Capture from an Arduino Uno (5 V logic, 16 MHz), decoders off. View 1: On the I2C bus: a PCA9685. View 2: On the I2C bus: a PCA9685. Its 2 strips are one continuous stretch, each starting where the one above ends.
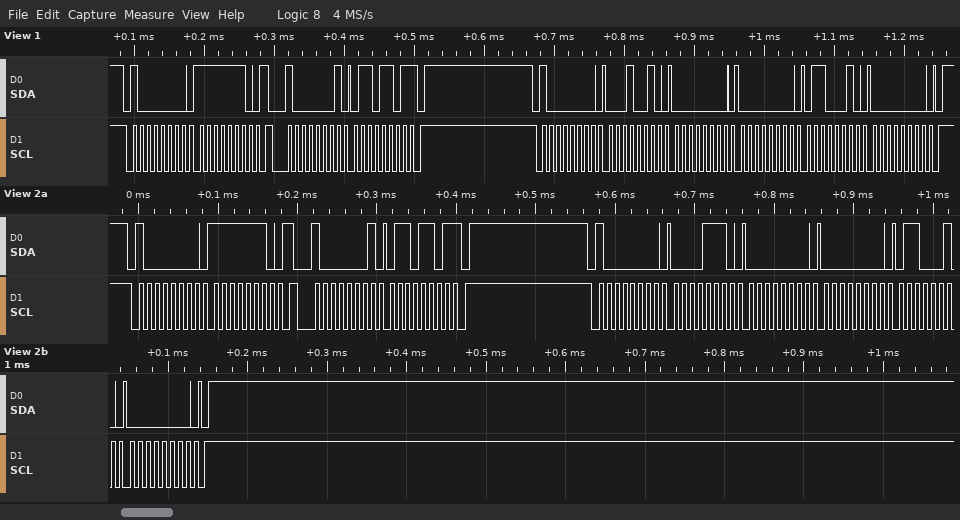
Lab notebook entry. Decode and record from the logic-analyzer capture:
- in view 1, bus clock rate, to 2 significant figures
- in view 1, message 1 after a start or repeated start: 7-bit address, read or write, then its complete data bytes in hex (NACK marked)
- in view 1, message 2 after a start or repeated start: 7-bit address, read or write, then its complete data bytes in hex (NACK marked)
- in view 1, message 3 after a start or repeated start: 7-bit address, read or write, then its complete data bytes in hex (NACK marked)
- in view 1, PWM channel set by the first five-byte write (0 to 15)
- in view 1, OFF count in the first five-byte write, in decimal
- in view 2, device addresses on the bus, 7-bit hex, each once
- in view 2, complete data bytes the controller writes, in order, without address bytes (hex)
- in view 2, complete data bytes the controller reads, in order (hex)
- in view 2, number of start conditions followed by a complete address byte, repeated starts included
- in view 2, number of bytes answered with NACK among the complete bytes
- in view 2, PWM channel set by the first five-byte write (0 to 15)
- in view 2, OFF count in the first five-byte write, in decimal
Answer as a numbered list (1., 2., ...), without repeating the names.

1. 100 kHz
2. 0x40 write: FE
3. 0x40 read: 6D NACK
4. 0x40 write: 12 00 00 62 00
5. 3
6. 98
7. 0x40
8. FE 0E 00 00 62 00
9. 6D
10. 3
11. 1
12. 2
13. 98
